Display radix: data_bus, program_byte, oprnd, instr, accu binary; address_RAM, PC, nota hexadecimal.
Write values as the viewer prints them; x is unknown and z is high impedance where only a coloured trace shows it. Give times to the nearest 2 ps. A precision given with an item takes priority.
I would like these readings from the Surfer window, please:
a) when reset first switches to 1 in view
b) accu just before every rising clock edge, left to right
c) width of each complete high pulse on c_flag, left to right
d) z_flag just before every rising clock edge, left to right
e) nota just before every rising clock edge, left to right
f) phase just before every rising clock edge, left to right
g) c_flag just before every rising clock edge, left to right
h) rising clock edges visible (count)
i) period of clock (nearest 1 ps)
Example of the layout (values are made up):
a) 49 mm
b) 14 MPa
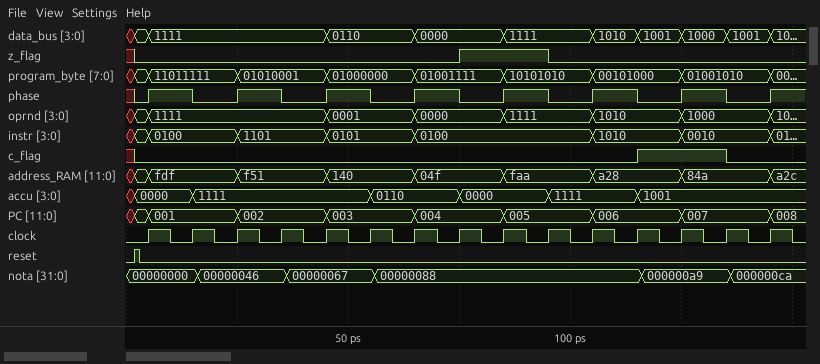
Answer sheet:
a) 2 ps
b) 0000, 0000, 1111, 1111, 1111, 1111, 0110, 0110, 0000, 0000, 1111, 1111, 1001, 1001, 1001
c) 20 ps
d) 0 0 0 0 0 0 0 0 1 1 0 0 0 0 0
e) 00000000, 00000000, 00000046, 00000046, 00000067, 00000067, 00000088, 00000088, 00000088, 00000088, 00000088, 00000088, 000000a9, 000000a9, 000000ca
f) 0 1 0 1 0 1 0 1 0 1 0 1 0 1 0
g) 0 0 0 0 0 0 0 0 0 0 0 0 1 1 0
h) 15
i) 10 ps
